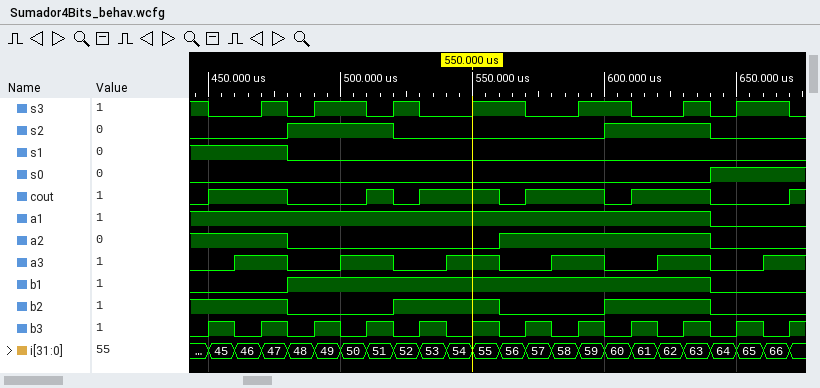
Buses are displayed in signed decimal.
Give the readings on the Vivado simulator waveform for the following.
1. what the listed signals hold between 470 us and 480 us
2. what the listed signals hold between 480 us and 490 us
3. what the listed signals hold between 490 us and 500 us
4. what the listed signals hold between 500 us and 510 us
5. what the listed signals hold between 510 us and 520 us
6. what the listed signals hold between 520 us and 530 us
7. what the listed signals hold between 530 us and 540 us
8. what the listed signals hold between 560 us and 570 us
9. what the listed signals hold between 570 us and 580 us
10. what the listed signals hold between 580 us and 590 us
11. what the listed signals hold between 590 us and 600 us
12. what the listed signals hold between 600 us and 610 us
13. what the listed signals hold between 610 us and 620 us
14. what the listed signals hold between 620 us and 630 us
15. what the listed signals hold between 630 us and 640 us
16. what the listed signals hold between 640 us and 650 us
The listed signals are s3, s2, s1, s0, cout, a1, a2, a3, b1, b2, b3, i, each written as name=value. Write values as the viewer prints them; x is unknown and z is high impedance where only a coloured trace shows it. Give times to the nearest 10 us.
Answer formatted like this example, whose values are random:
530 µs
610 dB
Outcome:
s3=1, s2=0, s1=1, s0=0, cout=1, a1=1, a2=1, a3=1, b1=0, b2=1, b3=1, i=47
s3=0, s2=1, s1=0, s0=0, cout=0, a1=1, a2=0, a3=0, b1=1, b2=0, b3=0, i=48
s3=1, s2=1, s1=0, s0=0, cout=0, a1=1, a2=0, a3=0, b1=1, b2=0, b3=1, i=49
s3=1, s2=1, s1=0, s0=0, cout=0, a1=1, a2=0, a3=1, b1=1, b2=0, b3=0, i=50
s3=0, s2=1, s1=0, s0=0, cout=1, a1=1, a2=0, a3=1, b1=1, b2=0, b3=1, i=51
s3=1, s2=0, s1=0, s0=0, cout=0, a1=1, a2=0, a3=0, b1=1, b2=1, b3=0, i=52
s3=0, s2=0, s1=0, s0=0, cout=1, a1=1, a2=0, a3=0, b1=1, b2=1, b3=1, i=53
s3=1, s2=0, s1=0, s0=0, cout=0, a1=1, a2=1, a3=0, b1=1, b2=0, b3=0, i=56
s3=0, s2=0, s1=0, s0=0, cout=1, a1=1, a2=1, a3=0, b1=1, b2=0, b3=1, i=57
s3=0, s2=0, s1=0, s0=0, cout=1, a1=1, a2=1, a3=1, b1=1, b2=0, b3=0, i=58
s3=1, s2=0, s1=0, s0=0, cout=1, a1=1, a2=1, a3=1, b1=1, b2=0, b3=1, i=59
s3=1, s2=1, s1=0, s0=0, cout=0, a1=1, a2=1, a3=0, b1=1, b2=1, b3=0, i=60
s3=0, s2=1, s1=0, s0=0, cout=1, a1=1, a2=1, a3=0, b1=1, b2=1, b3=1, i=61
s3=0, s2=1, s1=0, s0=0, cout=1, a1=1, a2=1, a3=1, b1=1, b2=1, b3=0, i=62
s3=1, s2=1, s1=0, s0=0, cout=1, a1=1, a2=1, a3=1, b1=1, b2=1, b3=1, i=63
s3=0, s2=0, s1=0, s0=1, cout=0, a1=0, a2=0, a3=0, b1=0, b2=0, b3=0, i=64
